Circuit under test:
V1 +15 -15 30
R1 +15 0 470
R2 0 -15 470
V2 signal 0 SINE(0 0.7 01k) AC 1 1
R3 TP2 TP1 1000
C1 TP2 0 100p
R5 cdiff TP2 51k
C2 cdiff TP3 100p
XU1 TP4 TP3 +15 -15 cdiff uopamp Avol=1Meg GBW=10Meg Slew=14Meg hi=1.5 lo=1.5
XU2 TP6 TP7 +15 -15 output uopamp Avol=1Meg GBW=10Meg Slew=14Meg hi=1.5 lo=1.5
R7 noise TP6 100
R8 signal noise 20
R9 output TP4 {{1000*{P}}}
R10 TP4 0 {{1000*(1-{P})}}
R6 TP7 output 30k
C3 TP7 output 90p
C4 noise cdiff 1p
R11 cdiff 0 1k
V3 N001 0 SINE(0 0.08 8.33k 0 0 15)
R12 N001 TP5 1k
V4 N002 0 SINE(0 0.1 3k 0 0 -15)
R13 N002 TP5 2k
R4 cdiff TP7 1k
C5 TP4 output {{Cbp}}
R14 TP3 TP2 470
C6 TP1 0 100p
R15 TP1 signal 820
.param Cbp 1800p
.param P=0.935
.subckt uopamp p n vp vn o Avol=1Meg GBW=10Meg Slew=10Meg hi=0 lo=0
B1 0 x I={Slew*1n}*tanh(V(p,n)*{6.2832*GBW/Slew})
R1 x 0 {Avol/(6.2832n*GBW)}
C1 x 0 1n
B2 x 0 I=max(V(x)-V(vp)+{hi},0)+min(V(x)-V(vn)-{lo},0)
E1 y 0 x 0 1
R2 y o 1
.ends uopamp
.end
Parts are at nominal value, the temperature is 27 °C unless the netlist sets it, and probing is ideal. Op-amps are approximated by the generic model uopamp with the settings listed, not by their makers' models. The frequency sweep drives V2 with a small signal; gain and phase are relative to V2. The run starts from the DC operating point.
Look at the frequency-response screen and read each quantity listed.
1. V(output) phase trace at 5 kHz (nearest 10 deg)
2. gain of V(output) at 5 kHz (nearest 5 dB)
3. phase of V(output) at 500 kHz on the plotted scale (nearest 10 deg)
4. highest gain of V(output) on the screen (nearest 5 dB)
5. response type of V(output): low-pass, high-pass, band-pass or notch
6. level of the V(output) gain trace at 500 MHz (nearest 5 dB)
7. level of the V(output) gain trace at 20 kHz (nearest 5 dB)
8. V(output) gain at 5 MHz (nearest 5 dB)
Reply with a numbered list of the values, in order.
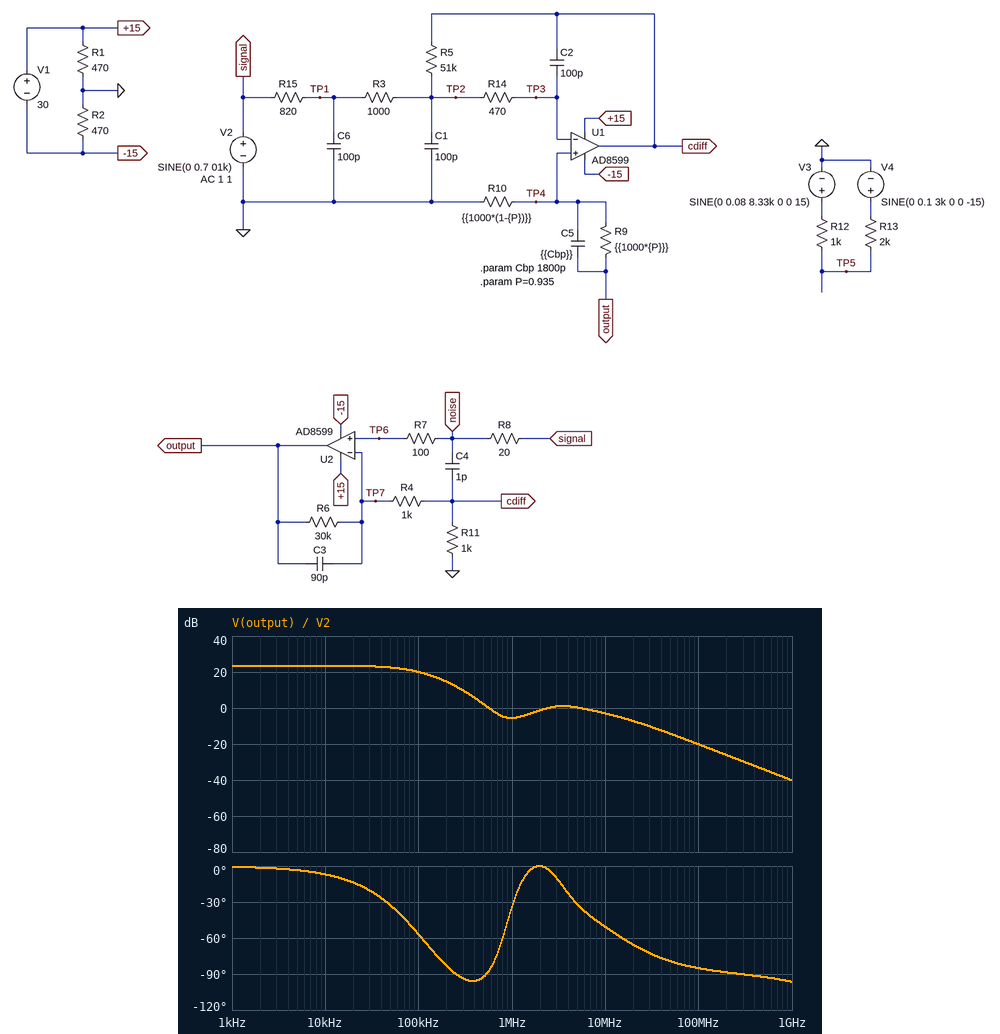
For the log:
1. 0 deg
2. 25 dB
3. -90 deg
4. 25 dB
5. low-pass
6. -35 dB
7. 25 dB
8. 0 dB
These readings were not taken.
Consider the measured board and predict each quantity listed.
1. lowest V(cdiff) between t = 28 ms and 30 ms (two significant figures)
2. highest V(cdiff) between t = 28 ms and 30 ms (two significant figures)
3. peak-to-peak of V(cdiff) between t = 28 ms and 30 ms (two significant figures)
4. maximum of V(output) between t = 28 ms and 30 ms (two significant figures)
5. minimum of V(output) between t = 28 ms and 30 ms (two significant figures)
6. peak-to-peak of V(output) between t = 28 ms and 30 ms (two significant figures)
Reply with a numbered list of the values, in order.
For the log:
1. -370 mV
2. 370 mV
3. 740 mV
4. 11 V
5. -11 V
6. 21 V
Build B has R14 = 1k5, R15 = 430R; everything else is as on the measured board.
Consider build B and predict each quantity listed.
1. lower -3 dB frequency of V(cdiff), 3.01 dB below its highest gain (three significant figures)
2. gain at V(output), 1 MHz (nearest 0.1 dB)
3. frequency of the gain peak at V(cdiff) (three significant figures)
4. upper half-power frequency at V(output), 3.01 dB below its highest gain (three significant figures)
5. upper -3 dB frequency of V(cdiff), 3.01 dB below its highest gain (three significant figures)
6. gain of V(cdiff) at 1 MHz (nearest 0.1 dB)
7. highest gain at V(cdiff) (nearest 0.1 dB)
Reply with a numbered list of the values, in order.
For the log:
1. 591 kHz
2. -3.1 dB
3. 2.69 MHz
4. 90.9 kHz
5. 6.66 MHz
6. -1.9 dB
7. -0.2 dB
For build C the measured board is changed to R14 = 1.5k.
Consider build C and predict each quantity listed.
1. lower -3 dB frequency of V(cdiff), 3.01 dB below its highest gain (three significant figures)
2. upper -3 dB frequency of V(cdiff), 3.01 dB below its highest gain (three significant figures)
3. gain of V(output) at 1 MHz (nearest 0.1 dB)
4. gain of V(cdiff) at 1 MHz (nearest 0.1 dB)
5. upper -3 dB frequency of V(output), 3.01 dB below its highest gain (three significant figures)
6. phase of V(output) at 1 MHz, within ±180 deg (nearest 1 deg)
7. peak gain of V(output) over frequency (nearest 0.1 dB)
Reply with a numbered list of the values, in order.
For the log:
1. 450 kHz
2. 6.68 MHz
3. -2.7 dB
4. -1.6 dB
5. 87.7 kHz
6. -27 deg
7. 23.6 dB
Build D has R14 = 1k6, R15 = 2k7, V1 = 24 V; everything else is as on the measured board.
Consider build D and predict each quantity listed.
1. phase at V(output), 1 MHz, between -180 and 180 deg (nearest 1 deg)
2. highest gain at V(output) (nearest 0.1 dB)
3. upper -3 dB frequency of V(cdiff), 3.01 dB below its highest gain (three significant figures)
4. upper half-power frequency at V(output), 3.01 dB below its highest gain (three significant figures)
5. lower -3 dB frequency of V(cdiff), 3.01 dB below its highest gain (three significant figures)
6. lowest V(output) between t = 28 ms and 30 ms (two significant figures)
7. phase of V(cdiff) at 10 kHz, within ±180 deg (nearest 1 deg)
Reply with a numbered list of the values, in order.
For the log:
1. -21 deg
2. 23.5 dB
3. 7.04 MHz
4. 72.7 kHz
5. 215 kHz
6. -10 V
7. -2 deg
